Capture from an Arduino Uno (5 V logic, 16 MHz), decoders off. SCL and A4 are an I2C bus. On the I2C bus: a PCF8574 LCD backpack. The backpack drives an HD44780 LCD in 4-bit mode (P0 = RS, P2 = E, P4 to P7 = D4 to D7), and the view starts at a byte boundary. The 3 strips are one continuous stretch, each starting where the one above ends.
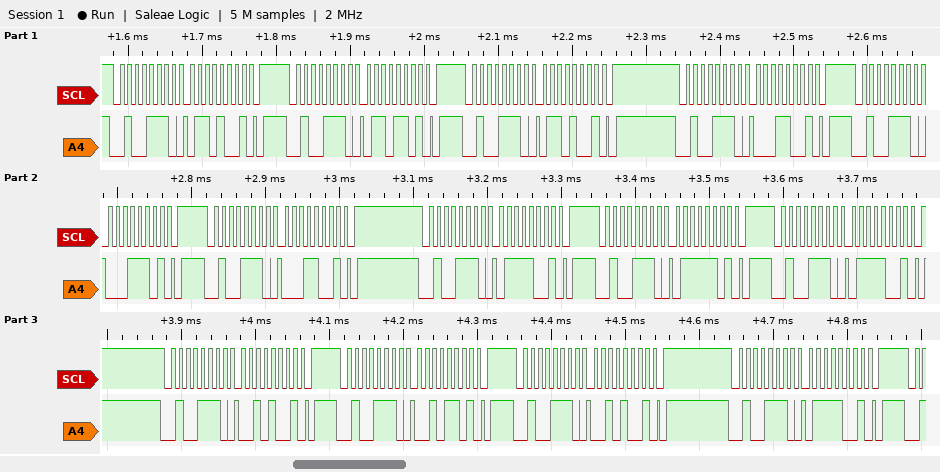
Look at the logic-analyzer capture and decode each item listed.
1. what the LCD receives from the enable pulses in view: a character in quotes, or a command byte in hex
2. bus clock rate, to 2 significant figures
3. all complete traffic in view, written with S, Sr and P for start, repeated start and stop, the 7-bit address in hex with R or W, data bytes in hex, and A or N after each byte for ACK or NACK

'a' 'r'
100 kHz
S 27W A 69 A P S 27W A 6D A P S 27W A 69 A P S 27W A 19 A P S 27W A 1D A P S 27W A 19 A P S 27W A 79 A P S 27W A 7D A P S 27W A 79 A P S 27W A 29 A P S 27W A 2D A P S 27W A 29 A P S 27W A 79 A P
